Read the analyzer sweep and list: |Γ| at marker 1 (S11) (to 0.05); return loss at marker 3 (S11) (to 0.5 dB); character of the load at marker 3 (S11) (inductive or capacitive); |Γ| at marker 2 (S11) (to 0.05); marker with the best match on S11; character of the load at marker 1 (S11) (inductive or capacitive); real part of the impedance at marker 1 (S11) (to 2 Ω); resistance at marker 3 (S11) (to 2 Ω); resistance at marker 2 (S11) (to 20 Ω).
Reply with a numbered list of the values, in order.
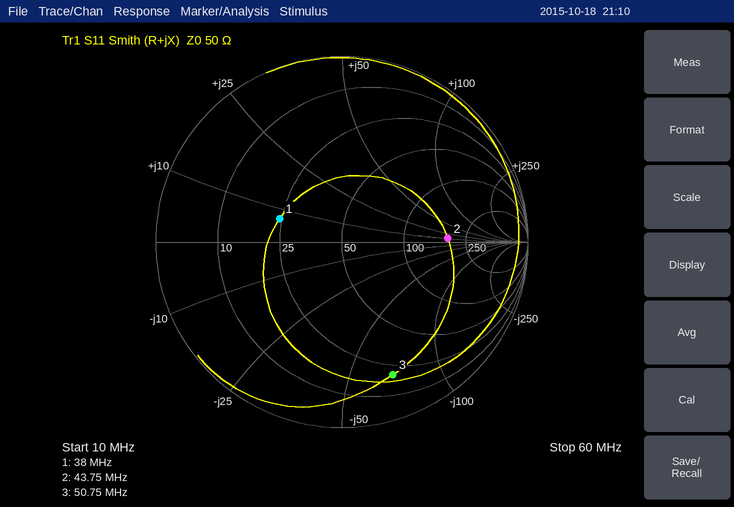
1. 0.35
2. 2.5 dB
3. capacitive
4. 0.55
5. marker 1
6. inductive
7. 24 Ω
8. 20 Ω
9. 180 Ω
